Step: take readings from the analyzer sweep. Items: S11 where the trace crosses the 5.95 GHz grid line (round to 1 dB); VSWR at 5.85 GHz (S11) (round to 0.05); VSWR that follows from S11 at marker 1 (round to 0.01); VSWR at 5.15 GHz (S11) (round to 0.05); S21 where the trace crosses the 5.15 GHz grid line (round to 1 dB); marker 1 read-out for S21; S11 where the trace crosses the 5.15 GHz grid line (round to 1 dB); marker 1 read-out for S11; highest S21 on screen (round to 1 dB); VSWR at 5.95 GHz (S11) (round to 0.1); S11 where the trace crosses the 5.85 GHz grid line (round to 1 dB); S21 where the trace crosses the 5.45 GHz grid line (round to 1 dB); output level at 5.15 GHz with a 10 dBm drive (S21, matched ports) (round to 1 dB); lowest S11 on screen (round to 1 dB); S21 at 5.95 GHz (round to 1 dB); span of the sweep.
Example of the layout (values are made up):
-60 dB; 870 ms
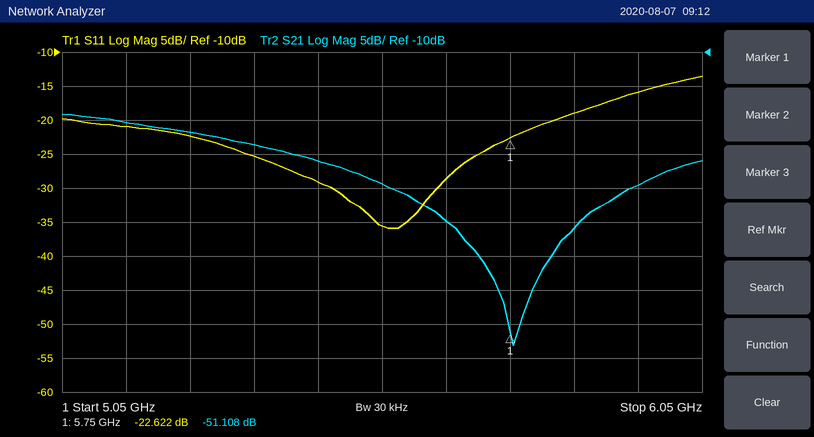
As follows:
-16 dB; 1.25; 1.16; 1.20; -20 dB; -51.108 dB; -21 dB; -22.622 dB; -19 dB; 1.4; -19 dB; -26 dB; -10 dBm; -36 dB; -30 dB; 1 GHz
